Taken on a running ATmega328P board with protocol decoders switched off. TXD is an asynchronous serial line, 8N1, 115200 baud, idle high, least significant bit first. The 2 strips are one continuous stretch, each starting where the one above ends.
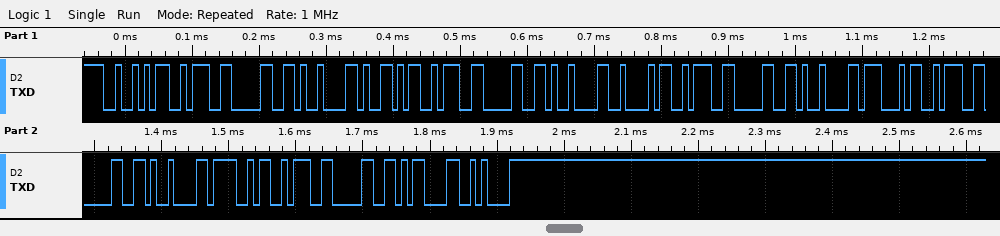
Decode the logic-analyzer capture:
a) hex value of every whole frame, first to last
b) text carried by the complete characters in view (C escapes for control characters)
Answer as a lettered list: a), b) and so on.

a) 52 3A 30 09 59 3A 30 09 42 3A 30 09 47 3A 30 09 4F 3A 30 0D 0A
b) "R:0\tY:0\tB:0\tG:0\tO:0\r\n"
